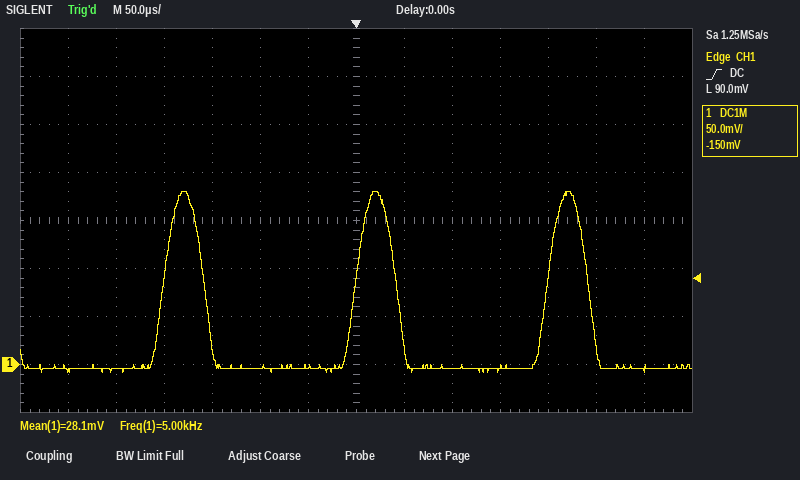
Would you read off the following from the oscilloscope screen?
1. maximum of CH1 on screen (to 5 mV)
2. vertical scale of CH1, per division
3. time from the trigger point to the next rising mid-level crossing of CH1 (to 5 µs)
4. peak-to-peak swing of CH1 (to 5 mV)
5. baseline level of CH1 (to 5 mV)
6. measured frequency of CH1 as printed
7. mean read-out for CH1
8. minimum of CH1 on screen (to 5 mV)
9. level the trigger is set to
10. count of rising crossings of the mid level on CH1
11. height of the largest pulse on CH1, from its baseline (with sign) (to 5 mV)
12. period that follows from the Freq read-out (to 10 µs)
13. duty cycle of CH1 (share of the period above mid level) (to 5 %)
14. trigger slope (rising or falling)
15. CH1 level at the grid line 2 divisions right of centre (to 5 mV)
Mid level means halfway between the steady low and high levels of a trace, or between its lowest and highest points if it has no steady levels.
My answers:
180 mV
50 mV
200 µs
190 mV
-5 mV
5.00 kHz
28.1 mV
-10 mV
90.0 mV
3
+185 mV
200 µs
20 %
rising
-5 mV
